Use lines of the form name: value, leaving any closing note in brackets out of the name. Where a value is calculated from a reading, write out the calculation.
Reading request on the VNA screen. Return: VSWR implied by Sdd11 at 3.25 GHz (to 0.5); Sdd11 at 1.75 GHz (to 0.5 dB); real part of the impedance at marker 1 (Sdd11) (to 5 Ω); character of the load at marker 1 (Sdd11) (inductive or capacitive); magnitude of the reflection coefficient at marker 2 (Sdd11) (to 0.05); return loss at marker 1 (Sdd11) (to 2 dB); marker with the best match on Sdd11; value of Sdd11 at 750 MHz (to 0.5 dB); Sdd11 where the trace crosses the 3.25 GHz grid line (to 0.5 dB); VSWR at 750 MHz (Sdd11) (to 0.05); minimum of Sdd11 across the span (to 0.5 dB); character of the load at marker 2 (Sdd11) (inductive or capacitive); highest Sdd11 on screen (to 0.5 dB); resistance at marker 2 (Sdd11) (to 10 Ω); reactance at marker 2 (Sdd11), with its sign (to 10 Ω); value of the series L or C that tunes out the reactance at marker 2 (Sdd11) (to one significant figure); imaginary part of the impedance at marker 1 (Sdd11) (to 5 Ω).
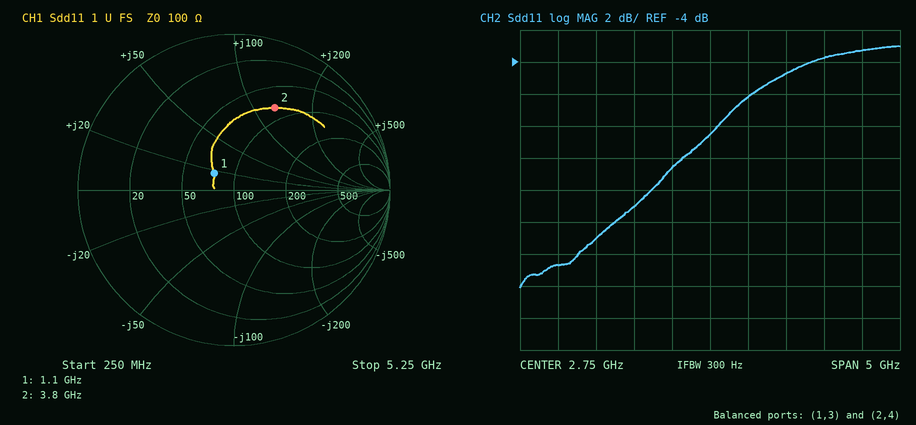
VSWR implied by Sdd11 at 3.25 GHz: |Γ| = 10^(-6/20) = 0.5012; VSWR = (1 + 0.5012)/(1 − 0.5012) ≈ 3.0
Sdd11 at 1.75 GHz: -13.0 dB
real part of the impedance at marker 1 (Sdd11): 75 Ω
character of the load at marker 1 (Sdd11): inductive
magnitude of the reflection coefficient at marker 2 (Sdd11): 0.60
return loss at marker 1 (Sdd11): 16 dB
marker with the best match on Sdd11: marker 1
value of Sdd11 at 750 MHz: -16.5 dB
Sdd11 where the trace crosses the 3.25 GHz grid line: -6.0 dB
VSWR at 750 MHz (Sdd11): |Γ| = 10^(-16.5/20) = 0.1496; VSWR = (1 + 0.1496)/(1 − 0.1496) ≈ 1.35
minimum of Sdd11 across the span: -18.0 dB
character of the load at marker 2 (Sdd11): inductive
highest Sdd11 on screen: -3.0 dB
resistance at marker 2 (Sdd11): 80 Ω
reactance at marker 2 (Sdd11), with its sign: +130 Ω
value of the series L or C that tunes out the reactance at marker 2 (Sdd11): C = 1/(2π × 3.8 GHz × 130 Ω) ≈ 322 fF, so 300 fF to one significant figure
imaginary part of the impedance at marker 1 (Sdd11): +15 Ω
